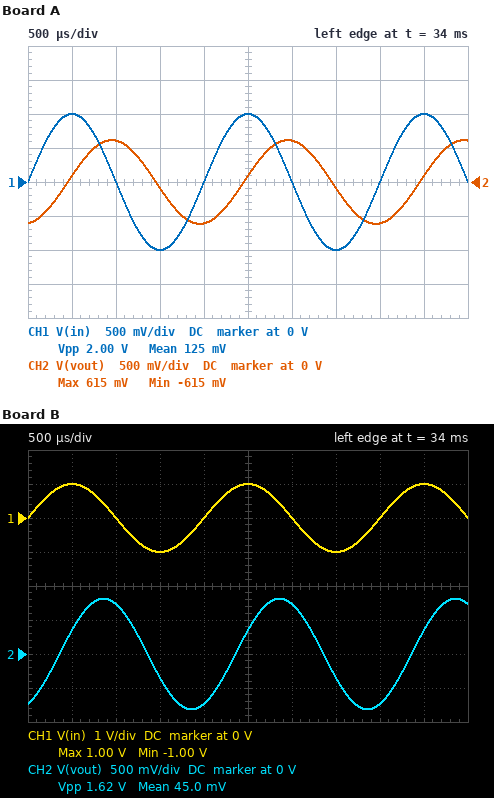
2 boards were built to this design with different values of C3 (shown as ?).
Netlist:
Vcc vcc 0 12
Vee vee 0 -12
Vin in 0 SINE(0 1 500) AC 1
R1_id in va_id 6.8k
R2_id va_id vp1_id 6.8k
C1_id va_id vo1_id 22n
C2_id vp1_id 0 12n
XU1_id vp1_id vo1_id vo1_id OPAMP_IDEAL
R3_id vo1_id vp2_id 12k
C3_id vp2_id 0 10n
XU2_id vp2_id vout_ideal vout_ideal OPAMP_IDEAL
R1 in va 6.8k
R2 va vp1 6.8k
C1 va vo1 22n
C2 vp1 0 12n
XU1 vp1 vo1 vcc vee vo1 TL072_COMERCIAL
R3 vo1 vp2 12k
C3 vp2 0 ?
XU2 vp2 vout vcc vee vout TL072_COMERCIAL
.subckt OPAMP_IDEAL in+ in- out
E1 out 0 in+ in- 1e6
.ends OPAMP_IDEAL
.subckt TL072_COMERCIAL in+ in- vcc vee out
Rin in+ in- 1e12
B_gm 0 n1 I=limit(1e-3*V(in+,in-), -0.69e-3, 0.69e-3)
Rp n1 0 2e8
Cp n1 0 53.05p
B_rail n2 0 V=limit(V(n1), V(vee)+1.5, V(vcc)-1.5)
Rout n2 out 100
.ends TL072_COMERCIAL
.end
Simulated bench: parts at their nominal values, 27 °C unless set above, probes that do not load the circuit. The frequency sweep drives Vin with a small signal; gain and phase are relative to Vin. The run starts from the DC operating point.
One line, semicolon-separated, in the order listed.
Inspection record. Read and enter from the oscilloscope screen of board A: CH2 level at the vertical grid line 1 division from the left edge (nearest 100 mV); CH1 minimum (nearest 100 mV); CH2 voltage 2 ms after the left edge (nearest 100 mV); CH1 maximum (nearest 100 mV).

100 mV; -1.0 V; -600 mV; 1.0 V
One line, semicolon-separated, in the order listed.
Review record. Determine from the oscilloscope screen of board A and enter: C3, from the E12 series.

33 nF
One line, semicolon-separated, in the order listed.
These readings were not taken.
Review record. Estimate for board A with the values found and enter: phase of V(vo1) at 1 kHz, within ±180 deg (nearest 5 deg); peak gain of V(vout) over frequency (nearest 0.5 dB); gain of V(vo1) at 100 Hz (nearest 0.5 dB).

-65 deg; 0 dB; 0 dB
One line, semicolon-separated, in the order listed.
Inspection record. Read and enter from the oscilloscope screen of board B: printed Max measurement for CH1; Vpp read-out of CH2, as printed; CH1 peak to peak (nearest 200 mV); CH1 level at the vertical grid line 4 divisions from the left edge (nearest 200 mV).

1.00 V; 1.62 V; 2.0 V; 0 V
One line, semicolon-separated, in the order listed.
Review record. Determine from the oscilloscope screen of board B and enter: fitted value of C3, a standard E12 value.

18 nF
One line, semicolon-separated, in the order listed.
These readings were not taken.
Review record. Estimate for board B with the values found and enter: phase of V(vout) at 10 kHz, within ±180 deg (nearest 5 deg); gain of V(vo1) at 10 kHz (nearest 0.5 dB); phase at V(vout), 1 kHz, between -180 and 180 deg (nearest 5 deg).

105 deg; -33.5 dB; -115 deg
